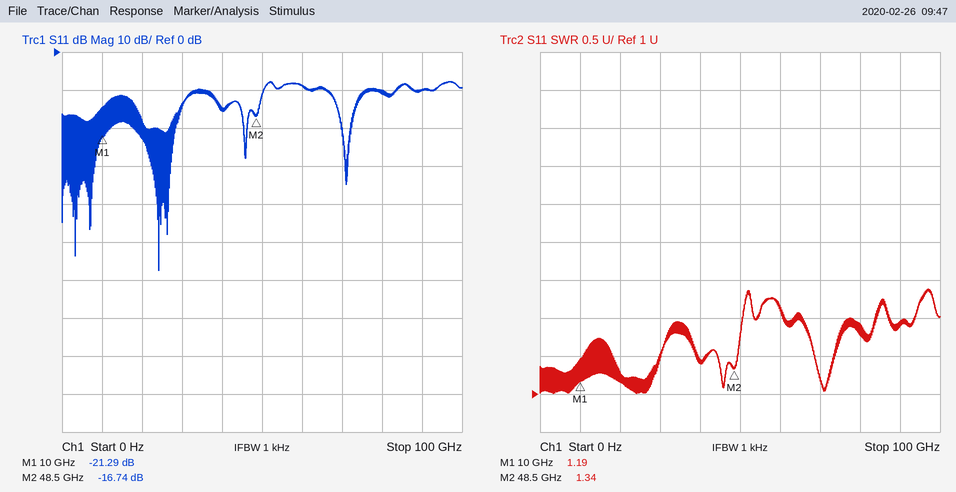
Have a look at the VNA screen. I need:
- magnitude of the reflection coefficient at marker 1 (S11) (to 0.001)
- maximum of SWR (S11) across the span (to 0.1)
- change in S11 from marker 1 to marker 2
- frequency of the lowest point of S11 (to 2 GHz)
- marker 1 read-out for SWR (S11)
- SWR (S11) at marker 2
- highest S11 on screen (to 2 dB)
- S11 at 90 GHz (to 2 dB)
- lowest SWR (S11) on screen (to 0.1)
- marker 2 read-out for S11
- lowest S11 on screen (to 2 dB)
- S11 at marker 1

0.086
2.4
4.55 dB
24 GHz
1.19
1.34
-8 dB
-10 dB
1.0
-16.74 dB
-58 dB
-21.29 dB
